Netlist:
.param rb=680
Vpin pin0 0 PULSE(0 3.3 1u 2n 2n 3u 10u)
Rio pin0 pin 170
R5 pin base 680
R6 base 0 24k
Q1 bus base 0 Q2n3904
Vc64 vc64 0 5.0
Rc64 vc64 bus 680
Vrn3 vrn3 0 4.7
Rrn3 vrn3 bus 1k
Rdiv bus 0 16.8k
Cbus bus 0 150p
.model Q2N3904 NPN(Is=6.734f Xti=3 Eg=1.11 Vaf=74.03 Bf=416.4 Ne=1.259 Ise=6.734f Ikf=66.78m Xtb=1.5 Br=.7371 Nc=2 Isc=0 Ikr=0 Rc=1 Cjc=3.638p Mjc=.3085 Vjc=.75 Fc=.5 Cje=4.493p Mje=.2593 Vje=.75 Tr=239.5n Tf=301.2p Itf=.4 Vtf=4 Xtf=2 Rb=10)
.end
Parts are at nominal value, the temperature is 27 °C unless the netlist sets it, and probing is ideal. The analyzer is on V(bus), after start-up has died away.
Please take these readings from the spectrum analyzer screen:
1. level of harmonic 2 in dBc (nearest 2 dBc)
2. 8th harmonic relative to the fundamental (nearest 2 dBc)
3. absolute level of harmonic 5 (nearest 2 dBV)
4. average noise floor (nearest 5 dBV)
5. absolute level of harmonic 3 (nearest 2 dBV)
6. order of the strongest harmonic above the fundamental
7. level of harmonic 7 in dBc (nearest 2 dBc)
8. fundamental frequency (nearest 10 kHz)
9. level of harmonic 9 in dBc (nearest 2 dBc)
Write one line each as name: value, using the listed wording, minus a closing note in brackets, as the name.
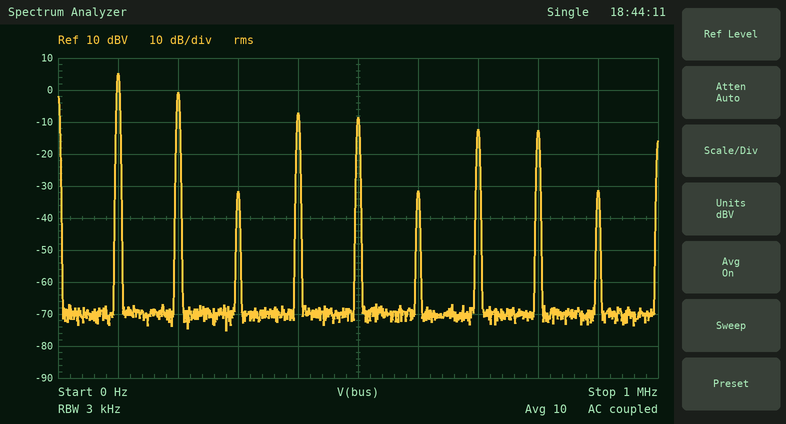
level of harmonic 2 in dBc: -6 dBc
8th harmonic relative to the fundamental: -18 dBc
absolute level of harmonic 5: -8 dBV
average noise floor: -70 dBV
absolute level of harmonic 3: -32 dBV
order of the strongest harmonic above the fundamental: 2
level of harmonic 7 in dBc: -18 dBc
fundamental frequency: 100 kHz
level of harmonic 9 in dBc: -36 dBc
